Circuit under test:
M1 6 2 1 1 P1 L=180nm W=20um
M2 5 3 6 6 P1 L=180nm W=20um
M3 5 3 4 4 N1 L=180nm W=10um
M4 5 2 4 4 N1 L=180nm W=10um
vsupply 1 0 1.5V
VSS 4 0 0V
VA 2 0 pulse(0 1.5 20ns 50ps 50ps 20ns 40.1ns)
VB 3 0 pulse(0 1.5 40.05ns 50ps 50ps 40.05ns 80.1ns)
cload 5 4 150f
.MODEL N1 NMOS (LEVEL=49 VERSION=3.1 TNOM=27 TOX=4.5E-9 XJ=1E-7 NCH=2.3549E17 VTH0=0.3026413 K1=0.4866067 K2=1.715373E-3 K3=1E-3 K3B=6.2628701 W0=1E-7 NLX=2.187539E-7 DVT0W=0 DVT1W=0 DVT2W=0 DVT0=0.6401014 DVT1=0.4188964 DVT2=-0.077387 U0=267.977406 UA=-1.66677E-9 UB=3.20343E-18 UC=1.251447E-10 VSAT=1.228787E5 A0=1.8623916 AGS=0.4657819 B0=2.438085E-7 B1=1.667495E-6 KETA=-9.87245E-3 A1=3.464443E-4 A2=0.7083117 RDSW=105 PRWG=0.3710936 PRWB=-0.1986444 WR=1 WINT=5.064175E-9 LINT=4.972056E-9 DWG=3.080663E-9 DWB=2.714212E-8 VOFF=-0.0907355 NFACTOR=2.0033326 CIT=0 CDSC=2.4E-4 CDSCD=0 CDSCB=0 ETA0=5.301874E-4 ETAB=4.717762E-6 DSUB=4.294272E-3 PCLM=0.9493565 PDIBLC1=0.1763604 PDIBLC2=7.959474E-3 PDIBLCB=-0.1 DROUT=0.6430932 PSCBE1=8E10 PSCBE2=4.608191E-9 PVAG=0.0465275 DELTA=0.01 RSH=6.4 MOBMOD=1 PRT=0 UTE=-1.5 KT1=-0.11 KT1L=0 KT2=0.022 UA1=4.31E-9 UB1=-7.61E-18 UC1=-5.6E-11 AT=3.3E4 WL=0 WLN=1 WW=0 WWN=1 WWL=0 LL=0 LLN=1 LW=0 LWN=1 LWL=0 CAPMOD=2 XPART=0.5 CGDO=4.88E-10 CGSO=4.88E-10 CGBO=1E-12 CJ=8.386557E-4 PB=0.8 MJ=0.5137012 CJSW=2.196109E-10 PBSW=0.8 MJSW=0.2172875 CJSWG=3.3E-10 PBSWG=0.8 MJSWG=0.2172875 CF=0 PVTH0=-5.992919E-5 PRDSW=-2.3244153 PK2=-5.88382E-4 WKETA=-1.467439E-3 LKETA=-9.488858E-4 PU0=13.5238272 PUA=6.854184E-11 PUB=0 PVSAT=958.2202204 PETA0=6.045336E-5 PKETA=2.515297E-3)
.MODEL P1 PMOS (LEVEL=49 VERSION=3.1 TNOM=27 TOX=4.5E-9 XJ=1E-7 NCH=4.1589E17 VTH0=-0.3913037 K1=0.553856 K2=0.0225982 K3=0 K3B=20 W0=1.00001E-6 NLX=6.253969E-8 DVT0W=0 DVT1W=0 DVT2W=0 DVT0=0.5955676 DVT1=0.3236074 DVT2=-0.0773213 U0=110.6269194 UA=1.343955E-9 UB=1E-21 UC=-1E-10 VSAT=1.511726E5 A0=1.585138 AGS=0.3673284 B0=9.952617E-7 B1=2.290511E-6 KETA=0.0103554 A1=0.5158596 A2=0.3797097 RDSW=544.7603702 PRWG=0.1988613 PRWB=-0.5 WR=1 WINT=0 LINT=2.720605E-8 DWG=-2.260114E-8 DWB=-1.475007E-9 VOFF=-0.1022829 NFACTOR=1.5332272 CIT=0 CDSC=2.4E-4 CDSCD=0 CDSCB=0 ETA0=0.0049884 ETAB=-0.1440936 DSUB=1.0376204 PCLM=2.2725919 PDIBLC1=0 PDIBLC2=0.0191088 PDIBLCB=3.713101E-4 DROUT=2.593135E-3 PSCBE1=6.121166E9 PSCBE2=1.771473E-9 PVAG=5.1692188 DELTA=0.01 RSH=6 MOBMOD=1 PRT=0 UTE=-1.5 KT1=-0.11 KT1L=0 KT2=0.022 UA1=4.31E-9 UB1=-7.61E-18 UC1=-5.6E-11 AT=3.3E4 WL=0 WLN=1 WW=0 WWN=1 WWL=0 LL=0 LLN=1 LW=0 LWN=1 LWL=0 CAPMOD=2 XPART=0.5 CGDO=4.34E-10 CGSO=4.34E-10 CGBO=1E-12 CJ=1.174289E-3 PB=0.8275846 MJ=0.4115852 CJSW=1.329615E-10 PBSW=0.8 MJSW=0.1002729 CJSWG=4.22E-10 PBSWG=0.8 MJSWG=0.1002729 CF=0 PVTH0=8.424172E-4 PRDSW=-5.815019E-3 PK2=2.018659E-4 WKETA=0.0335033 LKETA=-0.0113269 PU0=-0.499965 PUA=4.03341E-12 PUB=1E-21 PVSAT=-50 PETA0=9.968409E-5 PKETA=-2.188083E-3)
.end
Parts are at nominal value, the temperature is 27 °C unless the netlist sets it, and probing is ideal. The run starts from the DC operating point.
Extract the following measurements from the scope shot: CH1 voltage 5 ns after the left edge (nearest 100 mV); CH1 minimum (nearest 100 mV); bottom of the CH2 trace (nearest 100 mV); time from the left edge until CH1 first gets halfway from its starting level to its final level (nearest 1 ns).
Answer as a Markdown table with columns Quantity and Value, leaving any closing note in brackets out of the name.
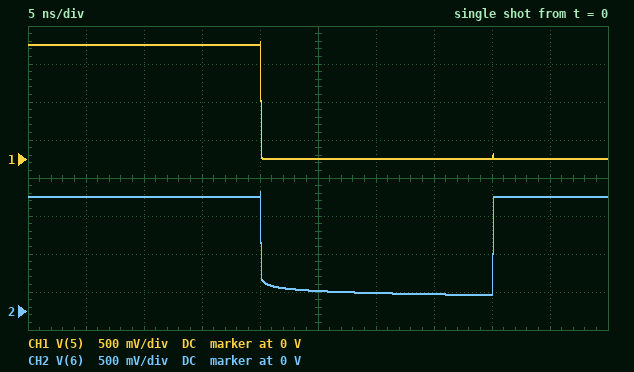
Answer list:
| Quantity | Value |
|---|---|
| CH1 voltage 5 ns after the left edge | 1.5 V |
| CH1 minimum | 0 V |
| bottom of the CH2 trace | 200 mV |
| time from the left edge until CH1 first gets halfway from its starting level to its final level | 20 ns |
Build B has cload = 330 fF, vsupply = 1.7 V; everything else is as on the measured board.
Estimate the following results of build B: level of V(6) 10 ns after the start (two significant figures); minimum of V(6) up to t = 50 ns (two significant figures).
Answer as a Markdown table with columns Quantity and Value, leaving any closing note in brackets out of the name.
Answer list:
| Quantity | Value |
|---|---|
| level of V(6) 10 ns after the start | 1.7 V |
| minimum of V(6) up to t = 50 ns | 230 mV |
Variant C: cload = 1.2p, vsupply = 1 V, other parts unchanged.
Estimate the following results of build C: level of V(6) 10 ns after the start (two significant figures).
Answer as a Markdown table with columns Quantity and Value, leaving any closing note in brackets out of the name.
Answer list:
| Quantity | Value |
|---|---|
| level of V(6) 10 ns after the start | 1.0 V |
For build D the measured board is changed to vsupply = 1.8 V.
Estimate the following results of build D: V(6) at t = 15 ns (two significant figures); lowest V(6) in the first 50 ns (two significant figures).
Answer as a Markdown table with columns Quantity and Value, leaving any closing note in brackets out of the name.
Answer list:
| Quantity | Value |
|---|---|
| V(6) at t = 15 ns | 1.8 V |
| lowest V(6) in the first 50 ns | 320 mV |
